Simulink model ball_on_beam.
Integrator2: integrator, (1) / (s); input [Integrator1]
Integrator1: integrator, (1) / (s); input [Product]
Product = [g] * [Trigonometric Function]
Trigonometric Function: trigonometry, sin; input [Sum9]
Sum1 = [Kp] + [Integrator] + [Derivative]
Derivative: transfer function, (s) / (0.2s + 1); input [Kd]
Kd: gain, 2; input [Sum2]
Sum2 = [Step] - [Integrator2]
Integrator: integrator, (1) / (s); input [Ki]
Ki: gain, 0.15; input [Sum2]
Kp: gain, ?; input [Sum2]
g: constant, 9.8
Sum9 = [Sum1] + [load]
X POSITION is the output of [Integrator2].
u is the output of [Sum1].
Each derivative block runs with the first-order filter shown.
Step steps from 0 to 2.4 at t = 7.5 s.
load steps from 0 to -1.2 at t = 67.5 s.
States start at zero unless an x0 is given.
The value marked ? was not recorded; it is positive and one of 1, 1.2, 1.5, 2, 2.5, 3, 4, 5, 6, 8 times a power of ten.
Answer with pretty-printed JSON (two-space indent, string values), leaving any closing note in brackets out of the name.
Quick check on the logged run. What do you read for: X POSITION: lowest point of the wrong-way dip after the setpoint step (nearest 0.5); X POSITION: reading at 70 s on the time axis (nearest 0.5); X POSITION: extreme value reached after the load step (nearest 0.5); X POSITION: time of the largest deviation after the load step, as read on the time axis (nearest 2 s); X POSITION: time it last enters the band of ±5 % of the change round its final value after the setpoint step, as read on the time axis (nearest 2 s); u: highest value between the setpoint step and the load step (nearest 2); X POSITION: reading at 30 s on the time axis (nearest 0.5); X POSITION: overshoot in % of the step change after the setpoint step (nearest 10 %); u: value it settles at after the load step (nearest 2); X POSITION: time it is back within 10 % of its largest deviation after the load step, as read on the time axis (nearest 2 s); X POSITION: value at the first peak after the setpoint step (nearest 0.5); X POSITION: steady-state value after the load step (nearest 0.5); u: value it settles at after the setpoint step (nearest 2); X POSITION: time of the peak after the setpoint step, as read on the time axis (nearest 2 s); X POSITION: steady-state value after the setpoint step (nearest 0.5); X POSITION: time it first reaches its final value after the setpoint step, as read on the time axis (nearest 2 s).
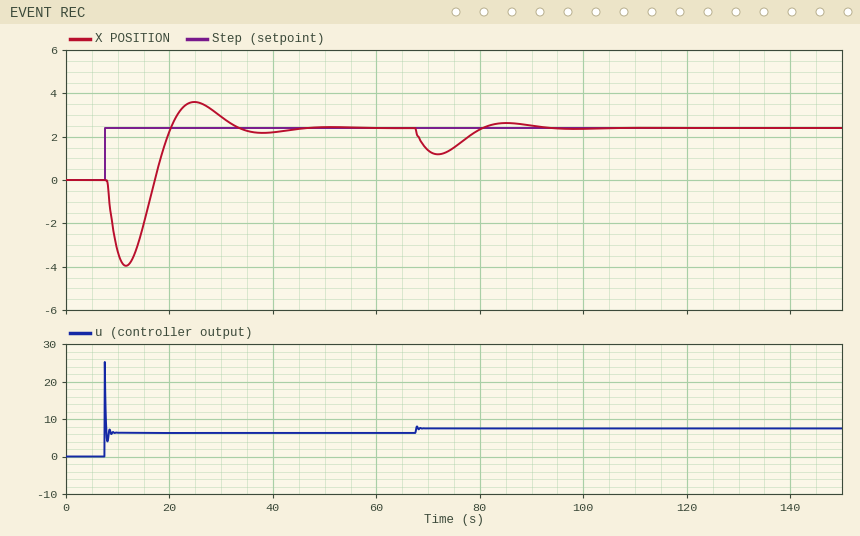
{
  "X POSITION: lowest point of the wrong-way dip after the setpoint step": "-4.0",
  "X POSITION: reading at 70 s on the time axis": "1.5",
  "X POSITION: extreme value reached after the load step": "1.0",
  "X POSITION: time of the largest deviation after the load step, as read on the time axis": "72 s",
  "X POSITION: time it last enters the band of ±5 % of the change round its final value after the setpoint step, as read on the time axis": "42 s",
  "u: highest value between the setpoint step and the load step": "26",
  "X POSITION: reading at 30 s on the time axis": "3.0",
  "X POSITION: overshoot in % of the step change after the setpoint step": "50 %",
  "u: value it settles at after the load step": "8",
  "X POSITION: time it is back within 10 % of its largest deviation after the load step, as read on the time axis": "90 s",
  "X POSITION: value at the first peak after the setpoint step": "3.5",
  "X POSITION: steady-state value after the load step": "2.5",
  "u: value it settles at after the setpoint step": "6",
  "X POSITION: time of the peak after the setpoint step, as read on the time axis": "24 s",
  "X POSITION: steady-state value after the setpoint step": "2.5",
  "X POSITION: time it first reaches its final value after the setpoint step, as read on the time axis": "20 s"
}
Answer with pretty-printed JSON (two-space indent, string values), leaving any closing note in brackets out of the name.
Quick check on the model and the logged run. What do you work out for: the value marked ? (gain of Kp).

{
  "the value marked ?": "0.5"
}
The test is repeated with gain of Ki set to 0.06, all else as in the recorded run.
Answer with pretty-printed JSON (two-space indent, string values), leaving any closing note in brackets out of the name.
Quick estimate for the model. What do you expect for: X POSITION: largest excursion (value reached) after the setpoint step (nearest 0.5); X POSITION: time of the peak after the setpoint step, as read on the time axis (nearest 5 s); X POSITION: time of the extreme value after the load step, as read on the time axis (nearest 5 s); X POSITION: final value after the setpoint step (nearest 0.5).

{
  "X POSITION: largest excursion (value reached) after the setpoint step": "2.5",
  "X POSITION: time of the peak after the setpoint step, as read on the time axis": "40 s",
  "X POSITION: time of the extreme value after the load step, as read on the time axis": "75 s",
  "X POSITION: final value after the setpoint step": "2.5"
}
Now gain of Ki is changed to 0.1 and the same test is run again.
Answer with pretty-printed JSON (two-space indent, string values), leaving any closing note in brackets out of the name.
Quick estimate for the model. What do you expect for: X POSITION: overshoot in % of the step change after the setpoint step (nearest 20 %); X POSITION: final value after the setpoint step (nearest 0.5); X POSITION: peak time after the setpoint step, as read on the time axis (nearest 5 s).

{
  "X POSITION: overshoot in % of the step change after the setpoint step": "40 %",
  "X POSITION: final value after the setpoint step": "2.5",
  "X POSITION: peak time after the setpoint step, as read on the time axis": "30 s"
}
